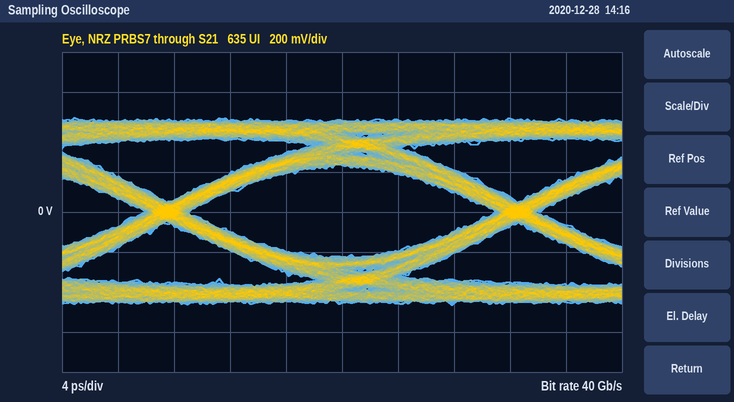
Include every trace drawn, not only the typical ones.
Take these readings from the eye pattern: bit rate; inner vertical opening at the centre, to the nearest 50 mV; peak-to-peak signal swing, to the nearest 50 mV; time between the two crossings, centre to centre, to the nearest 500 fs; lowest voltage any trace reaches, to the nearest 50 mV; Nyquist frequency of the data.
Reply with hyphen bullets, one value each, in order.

- 40 Gb/s
- 450 mV
- 950 mV
- 25.0 ps
- -450 mV
- 20 GHz
